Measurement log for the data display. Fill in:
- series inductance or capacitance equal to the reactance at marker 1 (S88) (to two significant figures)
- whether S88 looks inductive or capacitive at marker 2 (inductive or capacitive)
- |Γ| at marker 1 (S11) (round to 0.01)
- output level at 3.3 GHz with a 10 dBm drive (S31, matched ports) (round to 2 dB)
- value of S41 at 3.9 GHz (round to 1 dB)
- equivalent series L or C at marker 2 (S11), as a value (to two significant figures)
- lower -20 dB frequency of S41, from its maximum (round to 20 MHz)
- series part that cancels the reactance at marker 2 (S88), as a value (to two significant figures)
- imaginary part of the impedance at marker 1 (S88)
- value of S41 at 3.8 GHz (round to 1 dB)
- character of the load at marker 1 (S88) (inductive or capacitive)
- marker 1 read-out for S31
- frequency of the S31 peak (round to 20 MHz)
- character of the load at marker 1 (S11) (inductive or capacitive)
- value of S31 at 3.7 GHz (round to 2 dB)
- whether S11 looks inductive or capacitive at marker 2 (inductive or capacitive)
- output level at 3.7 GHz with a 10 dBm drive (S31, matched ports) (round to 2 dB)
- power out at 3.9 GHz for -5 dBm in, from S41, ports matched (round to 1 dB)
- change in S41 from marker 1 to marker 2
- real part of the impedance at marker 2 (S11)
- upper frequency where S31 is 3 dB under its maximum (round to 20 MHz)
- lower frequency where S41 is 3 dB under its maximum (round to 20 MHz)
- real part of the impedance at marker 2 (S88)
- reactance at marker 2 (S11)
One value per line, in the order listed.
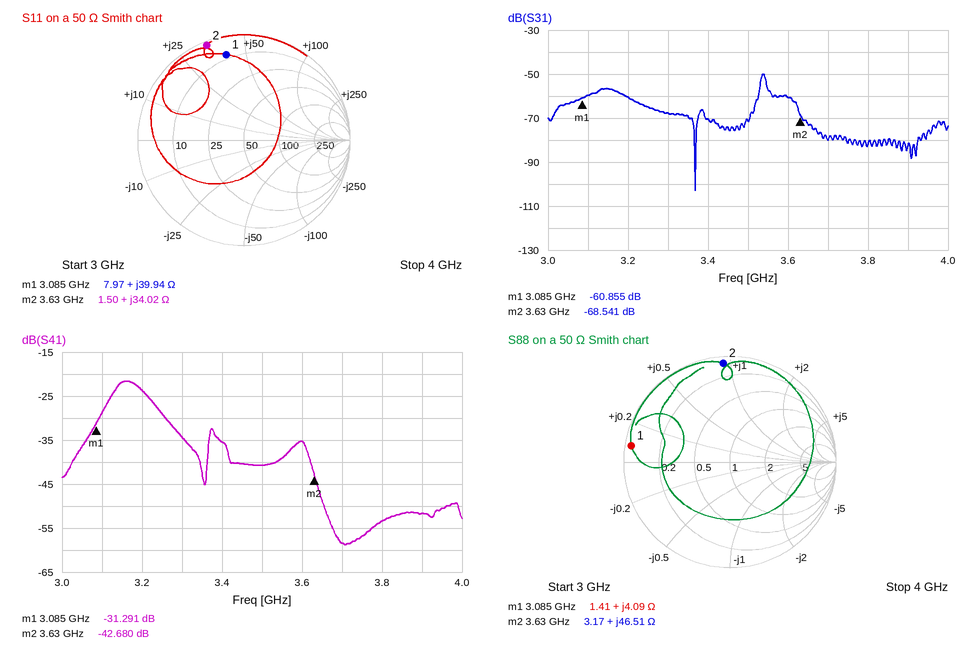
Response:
210 pH
inductive
0.82
-58 dBm
-52 dB
1.5 nH
3.02 GHz
940 fF
+4.09 Ω
-53 dB
inductive
-60.855 dB
3.54 GHz
inductive
-80 dB
inductive
-70 dBm
-57 dBm
-11.389 dB
1.50 Ω
3.54 GHz
3.12 GHz
3.17 Ω
+34.02 Ω
